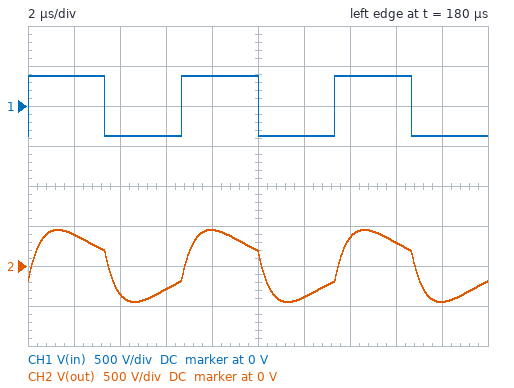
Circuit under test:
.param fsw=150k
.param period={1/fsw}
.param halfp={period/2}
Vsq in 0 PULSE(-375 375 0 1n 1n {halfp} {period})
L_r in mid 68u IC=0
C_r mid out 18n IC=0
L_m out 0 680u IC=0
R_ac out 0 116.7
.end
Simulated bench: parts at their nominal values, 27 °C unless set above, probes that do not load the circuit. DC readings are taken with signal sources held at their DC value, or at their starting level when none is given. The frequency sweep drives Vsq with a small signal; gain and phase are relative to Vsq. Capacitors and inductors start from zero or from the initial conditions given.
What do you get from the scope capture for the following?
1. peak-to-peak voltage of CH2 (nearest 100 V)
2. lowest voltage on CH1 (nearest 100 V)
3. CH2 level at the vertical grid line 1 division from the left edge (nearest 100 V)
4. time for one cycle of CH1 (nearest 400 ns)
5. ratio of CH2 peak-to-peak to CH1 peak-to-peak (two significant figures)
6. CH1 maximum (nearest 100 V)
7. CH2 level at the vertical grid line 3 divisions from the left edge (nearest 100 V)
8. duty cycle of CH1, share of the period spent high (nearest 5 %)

900 V
-400 V
400 V
6.8 µs
1.2
400 V
-300 V
50 %
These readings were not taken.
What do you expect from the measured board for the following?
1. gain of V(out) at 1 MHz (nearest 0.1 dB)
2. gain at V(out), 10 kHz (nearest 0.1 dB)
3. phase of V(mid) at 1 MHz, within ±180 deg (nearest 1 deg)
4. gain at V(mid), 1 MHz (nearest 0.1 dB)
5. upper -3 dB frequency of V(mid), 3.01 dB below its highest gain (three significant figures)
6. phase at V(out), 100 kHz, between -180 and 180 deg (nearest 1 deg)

-11.5 dB
-26.4 dB
-77 deg
-11.5 dB
256 kHz
24 deg
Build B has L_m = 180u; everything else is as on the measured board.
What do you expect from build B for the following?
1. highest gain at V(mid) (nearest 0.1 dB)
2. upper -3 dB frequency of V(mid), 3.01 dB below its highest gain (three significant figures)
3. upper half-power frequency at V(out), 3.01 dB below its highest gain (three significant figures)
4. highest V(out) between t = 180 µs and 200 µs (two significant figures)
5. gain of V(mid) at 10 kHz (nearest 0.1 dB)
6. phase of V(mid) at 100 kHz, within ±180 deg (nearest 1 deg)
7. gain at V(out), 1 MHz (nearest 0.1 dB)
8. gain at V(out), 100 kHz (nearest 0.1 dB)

3.4 dB
105 kHz
130 kHz
430 V
0 dB
-41 deg
-11.7 dB
2.9 dB
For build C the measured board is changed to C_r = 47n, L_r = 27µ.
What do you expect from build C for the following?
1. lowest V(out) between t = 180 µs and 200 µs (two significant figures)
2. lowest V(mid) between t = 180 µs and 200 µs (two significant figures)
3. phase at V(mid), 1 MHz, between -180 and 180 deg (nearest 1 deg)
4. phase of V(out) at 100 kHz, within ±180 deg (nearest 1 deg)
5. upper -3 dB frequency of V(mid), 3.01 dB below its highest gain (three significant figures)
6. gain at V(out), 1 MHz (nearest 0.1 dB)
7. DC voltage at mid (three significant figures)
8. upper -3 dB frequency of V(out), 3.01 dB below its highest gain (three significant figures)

-430 V
-380 V
-56 deg
9 deg
634 kHz
-4.9 dB
-375 V
481 kHz
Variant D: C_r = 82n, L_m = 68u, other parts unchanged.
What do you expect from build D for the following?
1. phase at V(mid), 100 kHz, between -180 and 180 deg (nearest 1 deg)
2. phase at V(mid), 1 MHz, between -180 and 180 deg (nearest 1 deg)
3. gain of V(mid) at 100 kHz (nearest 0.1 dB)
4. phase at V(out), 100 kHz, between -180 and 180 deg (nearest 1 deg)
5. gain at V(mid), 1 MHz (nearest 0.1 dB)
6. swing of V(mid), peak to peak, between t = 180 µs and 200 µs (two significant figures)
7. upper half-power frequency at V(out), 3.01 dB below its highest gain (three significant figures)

-24 deg
-62 deg
-8.7 dB
-7 deg
-12.4 dB
420 V
50.2 kHz
